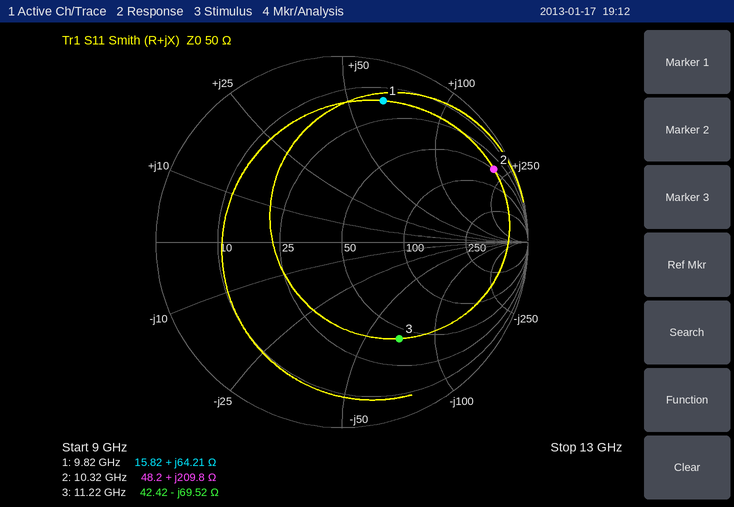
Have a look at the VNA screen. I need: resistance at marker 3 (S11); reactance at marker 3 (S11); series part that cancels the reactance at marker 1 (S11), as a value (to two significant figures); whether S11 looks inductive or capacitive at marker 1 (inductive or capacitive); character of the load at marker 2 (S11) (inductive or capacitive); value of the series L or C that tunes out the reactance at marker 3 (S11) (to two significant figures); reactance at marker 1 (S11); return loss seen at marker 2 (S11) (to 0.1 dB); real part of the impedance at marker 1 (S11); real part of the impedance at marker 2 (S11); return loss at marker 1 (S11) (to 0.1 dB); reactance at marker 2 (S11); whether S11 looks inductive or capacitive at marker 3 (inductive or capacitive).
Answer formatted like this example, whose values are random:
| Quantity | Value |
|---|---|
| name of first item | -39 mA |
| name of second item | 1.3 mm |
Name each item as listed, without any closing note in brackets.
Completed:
| Quantity | Value |
|---|---|
| resistance at marker 3 | 42.42 Ω |
| reactance at marker 3 | -69.52 Ω |
| series part that cancels the reactance at marker 1 (S11), as a value | 250 fF |
| whether S11 looks inductive or capacitive at marker 1 | inductive |
| character of the load at marker 2 (S11) | inductive |
| value of the series L or C that tunes out the reactance at marker 3 (S11) | 990 pH |
| reactance at marker 1 | +64.21 Ω |
| return loss seen at marker 2 (S11) | 0.9 dB |
| real part of the impedance at marker 1 | 15.82 Ω |
| real part of the impedance at marker 2 | 48.2 Ω |
| return loss at marker 1 (S11) | 2.0 dB |
| reactance at marker 2 | +209.8 Ω |
| whether S11 looks inductive or capacitive at marker 3 | capacitive |
